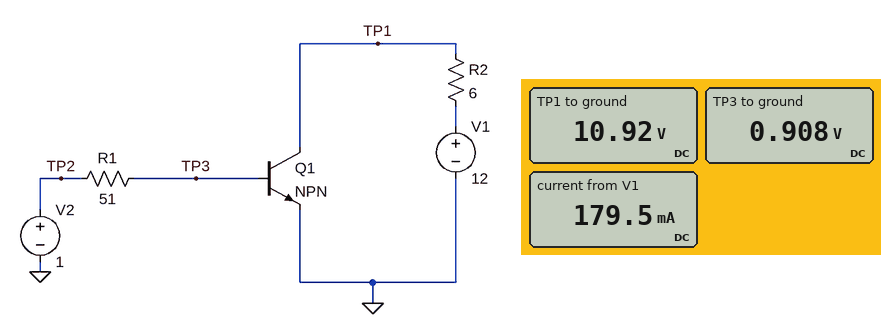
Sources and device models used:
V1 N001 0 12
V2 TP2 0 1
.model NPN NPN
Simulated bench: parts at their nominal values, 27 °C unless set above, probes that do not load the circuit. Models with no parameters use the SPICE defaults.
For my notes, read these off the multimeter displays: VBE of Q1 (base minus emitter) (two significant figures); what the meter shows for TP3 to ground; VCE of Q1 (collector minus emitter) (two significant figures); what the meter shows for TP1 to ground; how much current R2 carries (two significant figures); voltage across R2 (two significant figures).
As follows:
910 mV
0.908 V
11 V
10.92 V
180 mA
1.1 V
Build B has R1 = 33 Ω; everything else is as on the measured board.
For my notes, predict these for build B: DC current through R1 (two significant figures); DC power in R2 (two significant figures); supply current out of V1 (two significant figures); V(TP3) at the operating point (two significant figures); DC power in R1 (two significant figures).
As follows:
2.5 mA
380 mW
250 mA
920 mV
210 µW
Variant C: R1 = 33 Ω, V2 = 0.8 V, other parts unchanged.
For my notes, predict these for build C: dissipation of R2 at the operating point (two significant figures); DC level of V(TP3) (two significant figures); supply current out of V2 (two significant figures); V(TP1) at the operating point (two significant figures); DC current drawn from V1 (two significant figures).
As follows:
41 µW
800 mV
26 µA
12 V
2.6 mA
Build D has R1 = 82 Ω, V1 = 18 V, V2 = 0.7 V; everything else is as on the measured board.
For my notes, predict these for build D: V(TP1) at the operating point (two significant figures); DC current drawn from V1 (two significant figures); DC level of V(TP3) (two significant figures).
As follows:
18 V
57 µA
700 mV
